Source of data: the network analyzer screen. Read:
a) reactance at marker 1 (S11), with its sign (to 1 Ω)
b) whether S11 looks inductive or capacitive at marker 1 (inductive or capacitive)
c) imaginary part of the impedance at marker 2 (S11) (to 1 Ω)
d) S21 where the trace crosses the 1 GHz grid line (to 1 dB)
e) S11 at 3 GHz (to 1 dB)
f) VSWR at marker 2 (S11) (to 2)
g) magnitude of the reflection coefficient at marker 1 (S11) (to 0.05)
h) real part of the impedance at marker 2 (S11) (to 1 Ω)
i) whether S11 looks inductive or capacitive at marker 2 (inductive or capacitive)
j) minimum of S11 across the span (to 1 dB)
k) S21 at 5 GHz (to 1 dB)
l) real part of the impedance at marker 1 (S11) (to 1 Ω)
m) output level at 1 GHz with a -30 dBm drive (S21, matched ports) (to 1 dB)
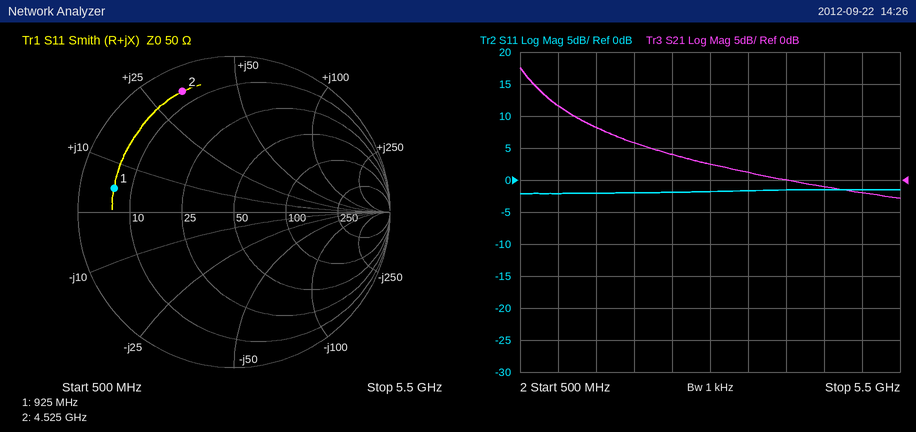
+5 Ω
inductive
+33 Ω
12 dB
-2 dB
12
0.80
6 Ω
inductive
-2 dB
-2 dB
6 Ω
-18 dBm
